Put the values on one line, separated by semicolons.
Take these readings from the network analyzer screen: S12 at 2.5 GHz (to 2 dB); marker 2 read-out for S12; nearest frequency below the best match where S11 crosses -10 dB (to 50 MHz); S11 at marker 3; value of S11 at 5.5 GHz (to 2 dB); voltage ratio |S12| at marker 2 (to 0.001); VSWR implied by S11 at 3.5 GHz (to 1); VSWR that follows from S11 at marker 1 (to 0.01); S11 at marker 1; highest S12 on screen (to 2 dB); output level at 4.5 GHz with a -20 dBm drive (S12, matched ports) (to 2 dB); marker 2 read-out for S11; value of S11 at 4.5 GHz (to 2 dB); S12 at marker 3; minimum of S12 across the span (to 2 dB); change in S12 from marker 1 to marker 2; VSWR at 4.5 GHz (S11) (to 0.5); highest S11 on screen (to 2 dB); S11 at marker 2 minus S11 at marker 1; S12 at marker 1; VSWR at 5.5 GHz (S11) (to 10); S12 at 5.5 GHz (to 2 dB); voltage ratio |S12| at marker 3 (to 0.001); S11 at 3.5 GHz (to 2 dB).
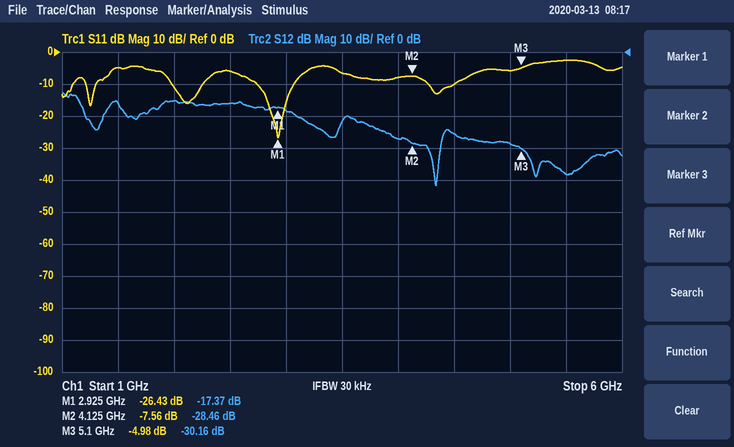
-16 dB; -28.46 dB; 2.75 GHz; -4.98 dB; -2 dB; 0.038; 3; 1.10; -26.43 dB; -12 dB; -46 dBm; -7.56 dB; -10 dB; -30.16 dB; -42 dB; -11.09 dB; 2.0; -2 dB; 18.87 dB; -17.37 dB; 10; -38 dB; 0.031; -6 dB
